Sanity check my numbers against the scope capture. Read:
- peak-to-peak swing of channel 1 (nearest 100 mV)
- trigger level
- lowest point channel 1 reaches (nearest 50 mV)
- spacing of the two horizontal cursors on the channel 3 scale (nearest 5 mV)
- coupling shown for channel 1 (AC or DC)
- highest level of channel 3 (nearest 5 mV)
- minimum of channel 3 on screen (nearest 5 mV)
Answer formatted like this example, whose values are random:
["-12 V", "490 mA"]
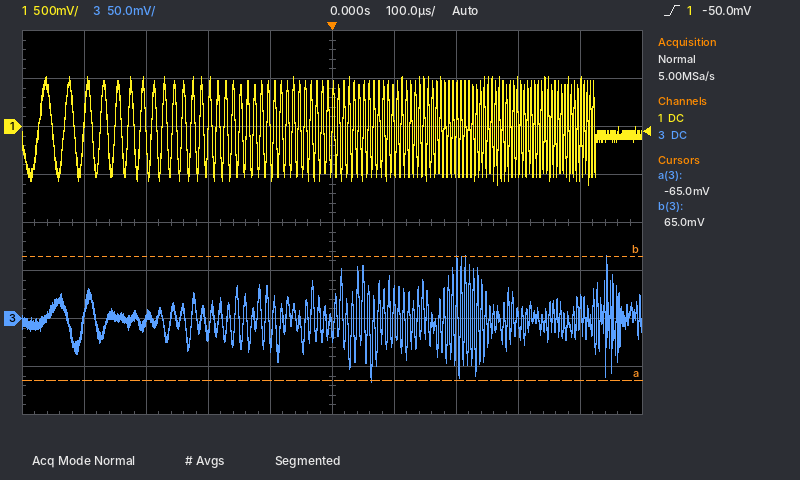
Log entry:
["1.10 V", "-50.0 mV", "-600 mV", "130 mV", "DC", "65 mV", "-65 mV"]
